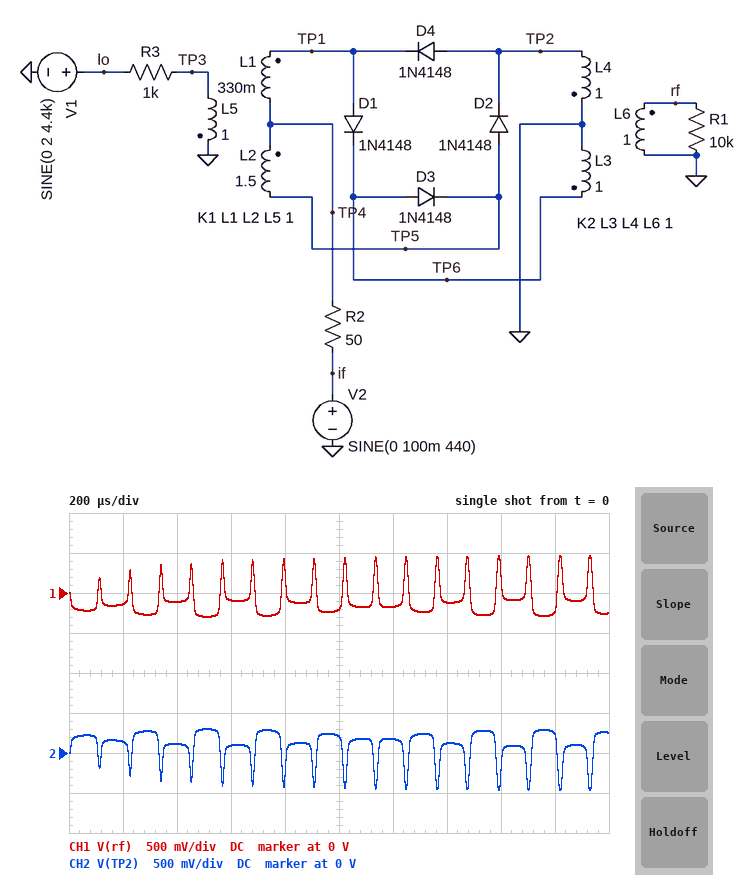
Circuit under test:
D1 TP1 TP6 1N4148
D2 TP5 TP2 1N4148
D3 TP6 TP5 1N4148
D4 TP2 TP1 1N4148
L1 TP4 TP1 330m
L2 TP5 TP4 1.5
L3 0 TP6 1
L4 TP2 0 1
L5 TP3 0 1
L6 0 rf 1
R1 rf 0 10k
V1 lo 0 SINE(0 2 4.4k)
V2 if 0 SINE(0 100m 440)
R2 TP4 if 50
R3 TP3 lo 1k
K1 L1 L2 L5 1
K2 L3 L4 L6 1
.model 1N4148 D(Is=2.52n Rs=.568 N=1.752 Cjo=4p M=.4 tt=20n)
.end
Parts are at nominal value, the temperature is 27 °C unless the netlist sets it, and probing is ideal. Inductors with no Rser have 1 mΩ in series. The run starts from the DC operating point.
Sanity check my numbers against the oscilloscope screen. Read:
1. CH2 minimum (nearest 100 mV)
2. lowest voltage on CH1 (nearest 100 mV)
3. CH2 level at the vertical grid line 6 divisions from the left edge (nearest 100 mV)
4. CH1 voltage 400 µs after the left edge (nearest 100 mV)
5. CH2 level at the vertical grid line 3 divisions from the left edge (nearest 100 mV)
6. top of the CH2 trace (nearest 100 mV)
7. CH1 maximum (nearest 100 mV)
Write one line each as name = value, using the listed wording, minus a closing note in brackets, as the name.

CH2 minimum = -500 mV
lowest voltage on CH1 = -300 mV
CH2 level at the vertical grid line 6 divisions from the left edge = 200 mV
CH1 voltage 400 µs after the left edge = -100 mV
CH2 level at the vertical grid line 3 divisions from the left edge = 100 mV
top of the CH2 trace = 300 mV
CH1 maximum = 500 mV
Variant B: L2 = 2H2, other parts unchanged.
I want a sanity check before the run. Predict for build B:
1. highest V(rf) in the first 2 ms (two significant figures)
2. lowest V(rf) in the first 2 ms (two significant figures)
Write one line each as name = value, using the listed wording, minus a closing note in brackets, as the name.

highest V(rf) in the first 2 ms = 480 mV
lowest V(rf) in the first 2 ms = -340 mV
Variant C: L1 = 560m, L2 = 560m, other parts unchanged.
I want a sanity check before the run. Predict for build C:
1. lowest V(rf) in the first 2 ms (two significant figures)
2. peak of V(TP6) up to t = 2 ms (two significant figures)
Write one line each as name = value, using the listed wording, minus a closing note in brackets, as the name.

lowest V(rf) in the first 2 ms = -99 mV
peak of V(TP6) up to t = 2 ms = 99 mV
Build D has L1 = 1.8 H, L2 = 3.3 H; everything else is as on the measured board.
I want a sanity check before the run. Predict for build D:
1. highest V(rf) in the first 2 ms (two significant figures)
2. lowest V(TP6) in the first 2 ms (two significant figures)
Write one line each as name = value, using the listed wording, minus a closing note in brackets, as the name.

highest V(rf) in the first 2 ms = 410 mV
lowest V(TP6) in the first 2 ms = -180 mV
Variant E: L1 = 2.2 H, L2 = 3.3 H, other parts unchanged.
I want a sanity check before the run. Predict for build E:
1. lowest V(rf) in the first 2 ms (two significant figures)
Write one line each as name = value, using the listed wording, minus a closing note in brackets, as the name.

lowest V(rf) in the first 2 ms = -150 mV
